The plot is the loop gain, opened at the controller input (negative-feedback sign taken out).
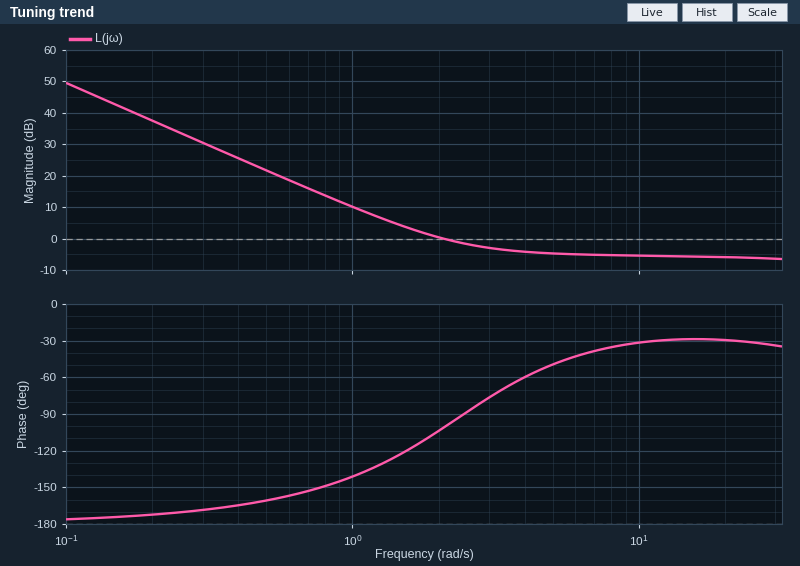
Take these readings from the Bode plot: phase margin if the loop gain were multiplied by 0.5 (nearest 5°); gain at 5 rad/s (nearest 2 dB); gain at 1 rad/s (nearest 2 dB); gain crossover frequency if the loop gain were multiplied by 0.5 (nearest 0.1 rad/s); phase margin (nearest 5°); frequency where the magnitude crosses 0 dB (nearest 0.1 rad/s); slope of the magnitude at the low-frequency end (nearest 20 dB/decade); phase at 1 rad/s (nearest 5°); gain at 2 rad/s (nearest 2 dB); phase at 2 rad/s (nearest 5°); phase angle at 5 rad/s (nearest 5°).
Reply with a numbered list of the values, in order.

1. 50°
2. -4 dB
3. 10 dB
4. 1.3 rad/s
5. 80°
6. 2.1 rad/s
7. -40 dB/decade
8. -140°
9. 0 dB
10. -105°
11. -50°
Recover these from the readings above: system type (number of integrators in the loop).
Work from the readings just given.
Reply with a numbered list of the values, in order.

1. 2
